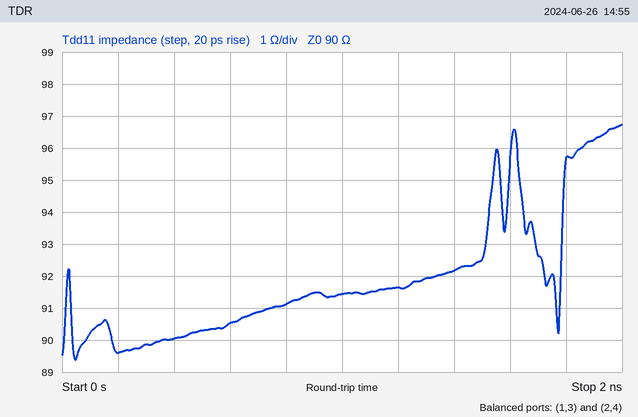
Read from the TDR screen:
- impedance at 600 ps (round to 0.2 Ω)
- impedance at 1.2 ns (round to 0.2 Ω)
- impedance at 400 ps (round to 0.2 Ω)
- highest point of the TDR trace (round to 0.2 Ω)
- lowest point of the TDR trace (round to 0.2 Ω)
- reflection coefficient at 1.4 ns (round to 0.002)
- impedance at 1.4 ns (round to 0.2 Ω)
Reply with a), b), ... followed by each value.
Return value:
a) 90.6 Ω
b) 91.6 Ω
c) 90.0 Ω
d) 96.8 Ω
e) 89.4 Ω
f) +0.012
g) 92.2 Ω
